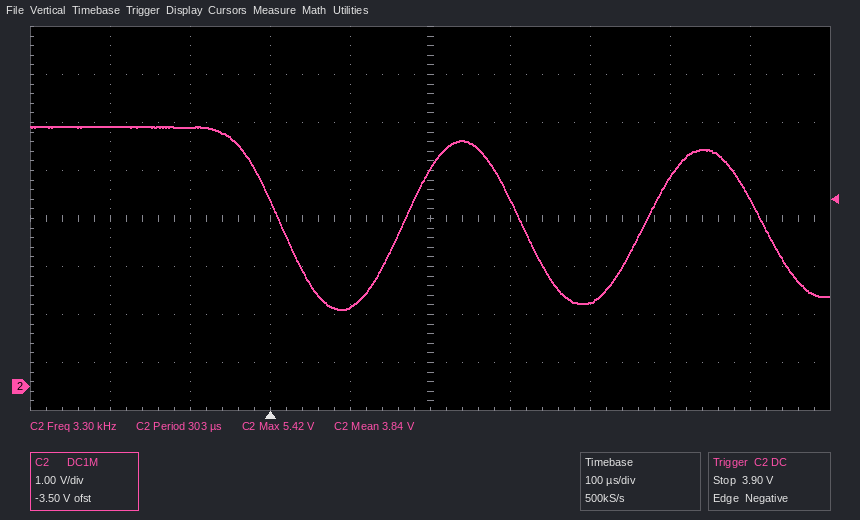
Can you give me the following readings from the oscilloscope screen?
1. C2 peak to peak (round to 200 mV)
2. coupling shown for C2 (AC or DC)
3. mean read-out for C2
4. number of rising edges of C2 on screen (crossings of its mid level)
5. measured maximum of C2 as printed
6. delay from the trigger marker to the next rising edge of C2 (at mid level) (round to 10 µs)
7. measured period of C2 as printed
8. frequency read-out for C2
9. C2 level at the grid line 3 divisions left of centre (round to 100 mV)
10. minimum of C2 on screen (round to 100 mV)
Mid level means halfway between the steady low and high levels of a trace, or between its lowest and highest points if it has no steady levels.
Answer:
3.8 V
DC
3.84 V
2
5.42 V
170 µs
303 µs
3.30 kHz
5.4 V
1.6 V
